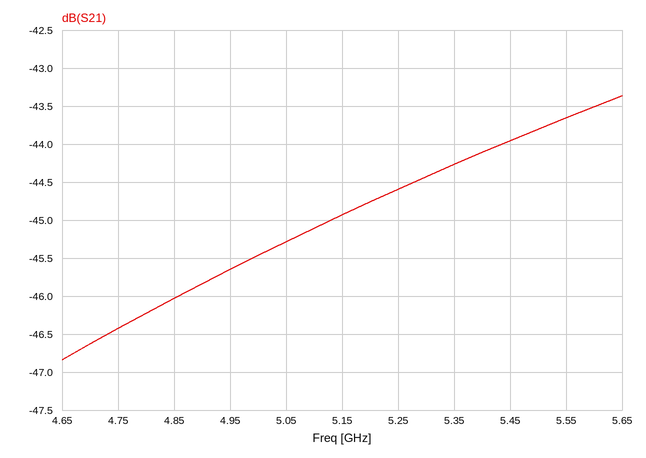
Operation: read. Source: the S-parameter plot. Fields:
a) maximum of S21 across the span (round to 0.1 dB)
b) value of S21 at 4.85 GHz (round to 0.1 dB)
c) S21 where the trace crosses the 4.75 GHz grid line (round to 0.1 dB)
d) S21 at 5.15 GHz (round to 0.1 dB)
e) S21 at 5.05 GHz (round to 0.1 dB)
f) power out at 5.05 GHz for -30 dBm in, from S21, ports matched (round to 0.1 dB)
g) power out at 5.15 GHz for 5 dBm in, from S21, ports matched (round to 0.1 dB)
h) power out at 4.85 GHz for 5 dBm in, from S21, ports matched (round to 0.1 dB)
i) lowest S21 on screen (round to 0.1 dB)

-43.4 dB
-46.0 dB
-46.4 dB
-44.9 dB
-45.3 dB
-75.3 dBm
-39.9 dBm
-41.0 dBm
-46.8 dB
